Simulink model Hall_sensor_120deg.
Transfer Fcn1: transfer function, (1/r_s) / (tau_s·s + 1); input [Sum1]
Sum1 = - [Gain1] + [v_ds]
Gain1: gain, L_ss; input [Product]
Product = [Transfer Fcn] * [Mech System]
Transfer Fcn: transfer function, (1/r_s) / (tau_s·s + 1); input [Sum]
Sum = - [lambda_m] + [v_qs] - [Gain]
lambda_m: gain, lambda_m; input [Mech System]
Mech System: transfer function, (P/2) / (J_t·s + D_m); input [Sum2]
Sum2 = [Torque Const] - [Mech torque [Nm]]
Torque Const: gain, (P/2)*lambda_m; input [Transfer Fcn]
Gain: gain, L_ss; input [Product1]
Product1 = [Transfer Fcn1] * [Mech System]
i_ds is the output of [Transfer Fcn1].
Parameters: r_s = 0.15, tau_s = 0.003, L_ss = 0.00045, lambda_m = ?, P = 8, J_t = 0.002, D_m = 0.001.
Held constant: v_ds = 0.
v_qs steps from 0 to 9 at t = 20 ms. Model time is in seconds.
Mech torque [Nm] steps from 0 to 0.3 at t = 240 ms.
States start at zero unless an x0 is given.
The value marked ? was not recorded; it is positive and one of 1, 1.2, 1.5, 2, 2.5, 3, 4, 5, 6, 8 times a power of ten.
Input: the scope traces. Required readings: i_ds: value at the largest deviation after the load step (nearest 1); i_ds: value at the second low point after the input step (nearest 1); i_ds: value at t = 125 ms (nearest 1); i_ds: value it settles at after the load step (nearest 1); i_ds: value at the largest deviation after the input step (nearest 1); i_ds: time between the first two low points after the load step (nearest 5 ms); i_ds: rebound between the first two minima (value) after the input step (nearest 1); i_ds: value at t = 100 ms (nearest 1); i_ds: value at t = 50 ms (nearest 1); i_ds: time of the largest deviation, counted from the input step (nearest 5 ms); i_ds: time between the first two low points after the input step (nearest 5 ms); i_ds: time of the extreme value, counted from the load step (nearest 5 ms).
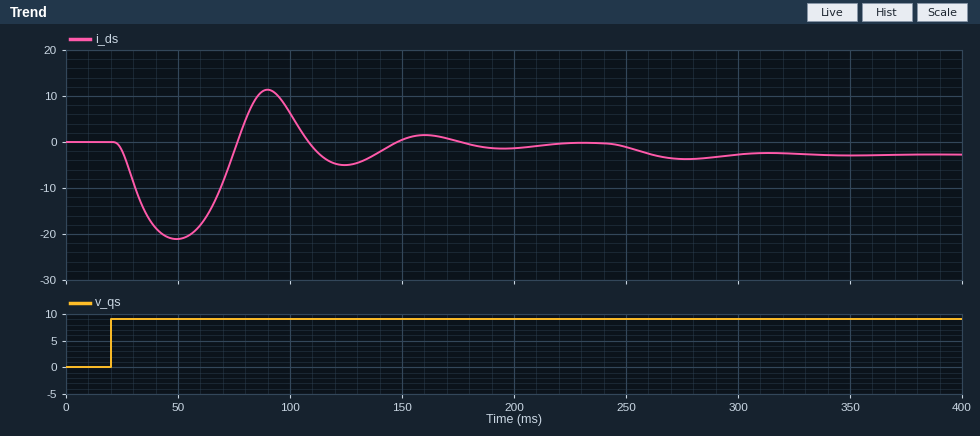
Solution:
-4
-5
-5
-3
-21
75 ms
11
6
-21
30 ms
75 ms
35 ms
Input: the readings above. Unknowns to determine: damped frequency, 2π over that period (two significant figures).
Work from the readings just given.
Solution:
0.084 rad/ms
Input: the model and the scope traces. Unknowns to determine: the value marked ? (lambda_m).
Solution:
0.03
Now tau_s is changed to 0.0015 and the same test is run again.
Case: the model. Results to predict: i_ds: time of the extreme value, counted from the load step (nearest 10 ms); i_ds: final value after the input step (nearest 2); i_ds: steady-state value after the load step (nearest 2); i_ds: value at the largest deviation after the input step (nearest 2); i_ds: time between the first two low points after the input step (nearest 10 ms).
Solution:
30 ms
0
-2
-20
60 ms
